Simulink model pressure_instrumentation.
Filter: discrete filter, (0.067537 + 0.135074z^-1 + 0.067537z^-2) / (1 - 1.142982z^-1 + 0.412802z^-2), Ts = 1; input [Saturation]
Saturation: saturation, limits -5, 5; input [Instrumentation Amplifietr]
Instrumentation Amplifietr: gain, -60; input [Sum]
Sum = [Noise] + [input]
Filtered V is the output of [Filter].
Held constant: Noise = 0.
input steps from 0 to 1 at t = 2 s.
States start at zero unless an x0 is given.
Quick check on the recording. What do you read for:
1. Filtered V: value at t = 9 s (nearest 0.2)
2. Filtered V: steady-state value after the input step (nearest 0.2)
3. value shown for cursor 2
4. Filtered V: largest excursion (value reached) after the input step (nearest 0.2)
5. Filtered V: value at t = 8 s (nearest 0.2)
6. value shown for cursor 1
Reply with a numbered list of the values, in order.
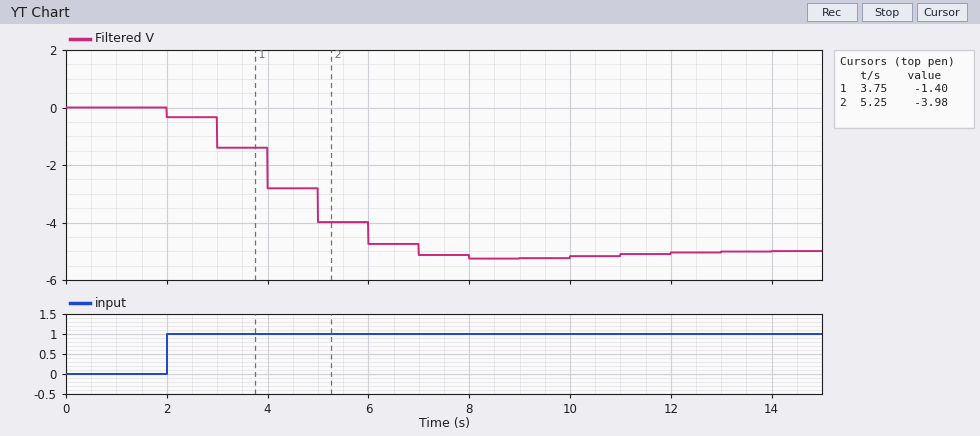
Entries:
1. -5.2
2. -5.0
3. -3.98
4. -5.2
5. -5.2
6. -1.40
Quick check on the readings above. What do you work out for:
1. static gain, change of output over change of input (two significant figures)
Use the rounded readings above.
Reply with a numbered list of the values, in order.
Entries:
1. -5.0
